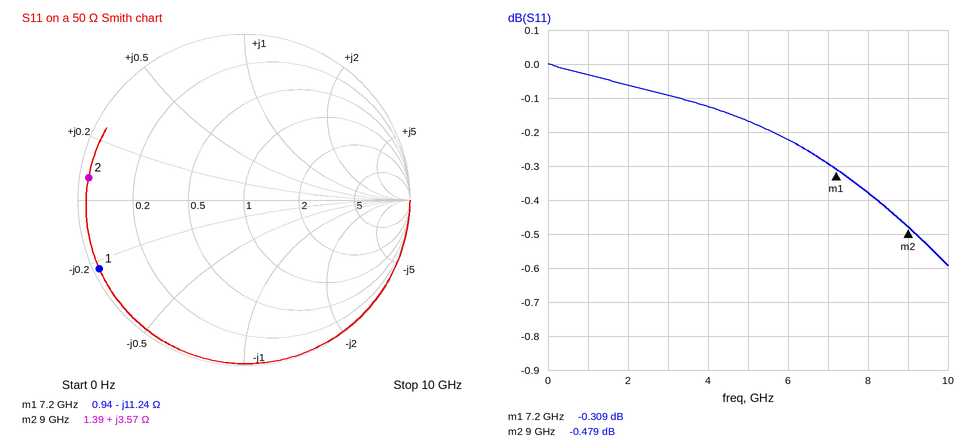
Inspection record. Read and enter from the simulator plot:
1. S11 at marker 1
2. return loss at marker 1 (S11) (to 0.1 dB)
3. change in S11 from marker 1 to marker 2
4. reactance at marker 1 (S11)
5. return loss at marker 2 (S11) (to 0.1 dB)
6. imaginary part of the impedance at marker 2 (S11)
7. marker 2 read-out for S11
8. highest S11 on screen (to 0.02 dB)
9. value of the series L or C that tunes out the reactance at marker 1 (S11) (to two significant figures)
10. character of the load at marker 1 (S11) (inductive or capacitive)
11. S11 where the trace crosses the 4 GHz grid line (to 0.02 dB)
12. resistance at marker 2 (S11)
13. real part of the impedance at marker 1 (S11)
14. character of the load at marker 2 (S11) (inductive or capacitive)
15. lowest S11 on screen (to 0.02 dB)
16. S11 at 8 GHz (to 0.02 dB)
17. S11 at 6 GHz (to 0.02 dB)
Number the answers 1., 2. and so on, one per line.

1. -0.309 dB
2. 0.3 dB
3. -0.170 dB
4. -11.24 Ω
5. 0.5 dB
6. +3.57 Ω
7. -0.479 dB
8. 0.00 dB
9. 250 pH
10. capacitive
11. -0.12 dB
12. 1.39 Ω
13. 0.94 Ω
14. inductive
15. -0.60 dB
16. -0.38 dB
17. -0.22 dB
